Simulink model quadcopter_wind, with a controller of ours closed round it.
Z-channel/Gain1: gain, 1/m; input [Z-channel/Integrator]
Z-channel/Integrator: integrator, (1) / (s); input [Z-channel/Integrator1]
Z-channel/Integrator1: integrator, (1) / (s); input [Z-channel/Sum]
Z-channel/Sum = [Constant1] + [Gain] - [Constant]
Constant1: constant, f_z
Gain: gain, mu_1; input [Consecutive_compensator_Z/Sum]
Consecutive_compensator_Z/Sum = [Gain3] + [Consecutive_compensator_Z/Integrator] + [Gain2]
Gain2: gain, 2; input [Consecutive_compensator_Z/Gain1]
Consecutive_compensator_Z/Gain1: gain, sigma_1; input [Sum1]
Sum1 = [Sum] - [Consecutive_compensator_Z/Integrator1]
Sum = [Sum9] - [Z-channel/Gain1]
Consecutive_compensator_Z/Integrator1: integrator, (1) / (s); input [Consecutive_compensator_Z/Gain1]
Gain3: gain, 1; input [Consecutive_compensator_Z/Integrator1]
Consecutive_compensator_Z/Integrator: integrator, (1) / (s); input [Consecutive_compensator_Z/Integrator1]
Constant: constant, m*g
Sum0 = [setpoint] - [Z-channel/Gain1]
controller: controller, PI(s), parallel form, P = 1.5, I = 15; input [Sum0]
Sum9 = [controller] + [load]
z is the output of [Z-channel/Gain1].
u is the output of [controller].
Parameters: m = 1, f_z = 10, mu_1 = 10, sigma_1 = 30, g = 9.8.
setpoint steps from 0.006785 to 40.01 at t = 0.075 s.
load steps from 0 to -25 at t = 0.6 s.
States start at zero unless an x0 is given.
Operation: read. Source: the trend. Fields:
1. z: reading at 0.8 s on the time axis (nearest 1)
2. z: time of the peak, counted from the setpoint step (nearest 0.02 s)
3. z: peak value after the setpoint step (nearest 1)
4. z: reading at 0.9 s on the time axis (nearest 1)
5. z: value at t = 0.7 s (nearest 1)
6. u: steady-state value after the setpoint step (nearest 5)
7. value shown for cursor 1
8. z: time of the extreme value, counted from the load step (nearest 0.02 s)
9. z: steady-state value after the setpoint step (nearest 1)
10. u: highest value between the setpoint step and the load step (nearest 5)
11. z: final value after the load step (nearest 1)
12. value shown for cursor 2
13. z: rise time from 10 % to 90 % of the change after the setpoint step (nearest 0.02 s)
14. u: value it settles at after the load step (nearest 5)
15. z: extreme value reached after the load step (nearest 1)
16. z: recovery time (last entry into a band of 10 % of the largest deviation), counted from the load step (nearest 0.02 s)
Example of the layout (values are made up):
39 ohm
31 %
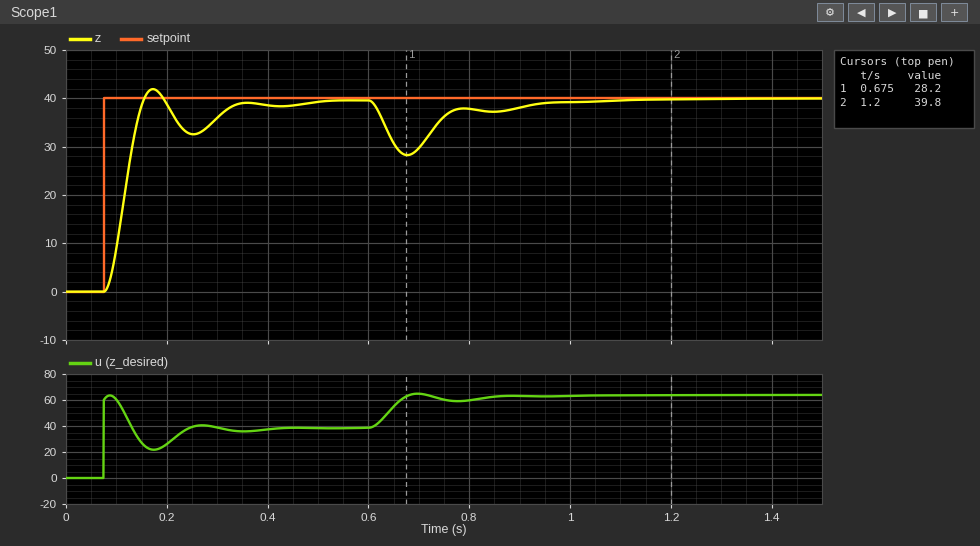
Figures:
38
0.10 s
42
38
30
40
28.2
0.08 s
40
65
40
39.8
0.06 s
65
28
0.34 s
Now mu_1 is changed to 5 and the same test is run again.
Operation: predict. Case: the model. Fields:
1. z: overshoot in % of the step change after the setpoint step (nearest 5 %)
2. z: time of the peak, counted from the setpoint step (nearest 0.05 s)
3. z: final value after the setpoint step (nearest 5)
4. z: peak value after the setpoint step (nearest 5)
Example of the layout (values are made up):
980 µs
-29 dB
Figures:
10 %
0.15 s
40
45
